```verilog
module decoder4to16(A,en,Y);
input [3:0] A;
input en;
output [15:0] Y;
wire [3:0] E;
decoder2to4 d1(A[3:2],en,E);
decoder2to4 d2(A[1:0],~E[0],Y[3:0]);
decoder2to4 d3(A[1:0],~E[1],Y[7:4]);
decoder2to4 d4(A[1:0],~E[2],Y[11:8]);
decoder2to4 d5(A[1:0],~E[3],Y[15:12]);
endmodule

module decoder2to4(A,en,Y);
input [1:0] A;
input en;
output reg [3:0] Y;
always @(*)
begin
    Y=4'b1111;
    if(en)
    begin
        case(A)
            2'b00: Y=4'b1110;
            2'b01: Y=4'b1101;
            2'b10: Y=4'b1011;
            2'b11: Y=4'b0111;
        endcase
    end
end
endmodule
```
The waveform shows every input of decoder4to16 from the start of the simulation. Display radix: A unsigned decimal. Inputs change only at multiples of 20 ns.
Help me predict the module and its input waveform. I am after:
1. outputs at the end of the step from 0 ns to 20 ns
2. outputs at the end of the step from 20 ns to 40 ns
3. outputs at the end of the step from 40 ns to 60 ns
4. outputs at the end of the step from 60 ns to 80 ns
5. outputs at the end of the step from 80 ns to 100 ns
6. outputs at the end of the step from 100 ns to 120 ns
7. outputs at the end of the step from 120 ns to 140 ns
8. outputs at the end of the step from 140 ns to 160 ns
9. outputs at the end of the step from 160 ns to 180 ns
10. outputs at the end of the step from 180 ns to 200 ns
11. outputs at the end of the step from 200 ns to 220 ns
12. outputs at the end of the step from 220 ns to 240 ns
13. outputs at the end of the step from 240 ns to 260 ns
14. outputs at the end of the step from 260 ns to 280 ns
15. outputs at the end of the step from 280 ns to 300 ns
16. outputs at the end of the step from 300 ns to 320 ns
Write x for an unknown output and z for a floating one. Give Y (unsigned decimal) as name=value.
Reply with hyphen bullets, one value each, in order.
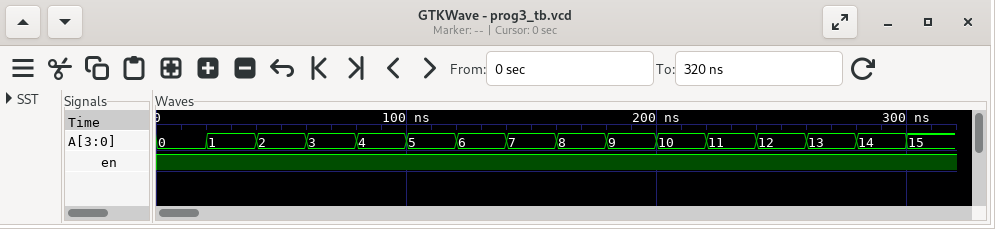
- Y=65534
- Y=65533
- Y=65531
- Y=65527
- Y=65519
- Y=65503
- Y=65471
- Y=65407
- Y=65279
- Y=65023
- Y=64511
- Y=63487
- Y=61439
- Y=57343
- Y=49151
- Y=32767
